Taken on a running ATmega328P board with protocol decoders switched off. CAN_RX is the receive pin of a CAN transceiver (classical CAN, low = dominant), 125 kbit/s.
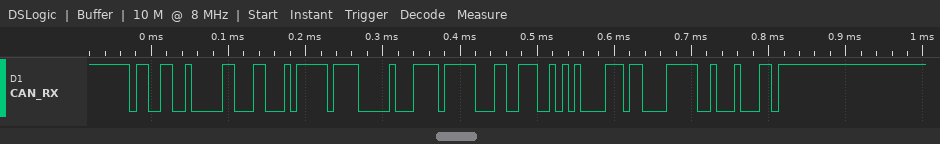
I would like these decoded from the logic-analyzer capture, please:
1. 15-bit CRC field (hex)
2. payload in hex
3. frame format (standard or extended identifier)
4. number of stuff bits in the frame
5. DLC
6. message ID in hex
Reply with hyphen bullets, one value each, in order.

- 0x7D11
- C5 FF 00 F7 CC E5 43 B0
- standard
- 5
- 8
- 0x664
